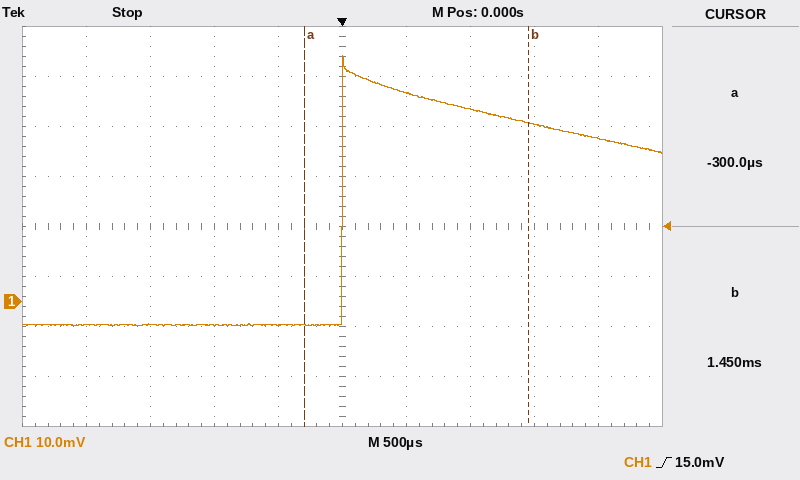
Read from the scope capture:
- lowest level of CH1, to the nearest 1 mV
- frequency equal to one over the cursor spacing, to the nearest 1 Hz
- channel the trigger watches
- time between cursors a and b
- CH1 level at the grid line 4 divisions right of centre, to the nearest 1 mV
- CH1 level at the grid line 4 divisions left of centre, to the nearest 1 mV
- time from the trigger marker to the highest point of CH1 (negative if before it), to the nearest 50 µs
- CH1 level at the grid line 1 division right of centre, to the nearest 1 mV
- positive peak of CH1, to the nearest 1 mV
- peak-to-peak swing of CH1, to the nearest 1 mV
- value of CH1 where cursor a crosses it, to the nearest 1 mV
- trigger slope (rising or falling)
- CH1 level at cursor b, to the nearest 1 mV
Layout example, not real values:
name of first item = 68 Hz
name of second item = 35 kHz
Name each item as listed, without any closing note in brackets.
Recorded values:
lowest level of CH1, to the nearest 1 mV = -5 mV
frequency equal to one over the cursor spacing, to the nearest 1 Hz = 571 Hz
channel the trigger watches = CH1
time between cursors a and b = 1.75 ms
CH1 level at the grid line 4 divisions right of centre, to the nearest 1 mV = 33 mV
CH1 level at the grid line 4 divisions left of centre, to the nearest 1 mV = -5 mV
time from the trigger marker to the highest point of CH1 (negative if before it), to the nearest 50 µs = 0 µs
CH1 level at the grid line 1 division right of centre, to the nearest 1 mV = 42 mV
positive peak of CH1, to the nearest 1 mV = 49 mV
peak-to-peak swing of CH1, to the nearest 1 mV = 54 mV
value of CH1 where cursor a crosses it, to the nearest 1 mV = -5 mV
trigger slope = rising
CH1 level at cursor b, to the nearest 1 mV = 36 mV
